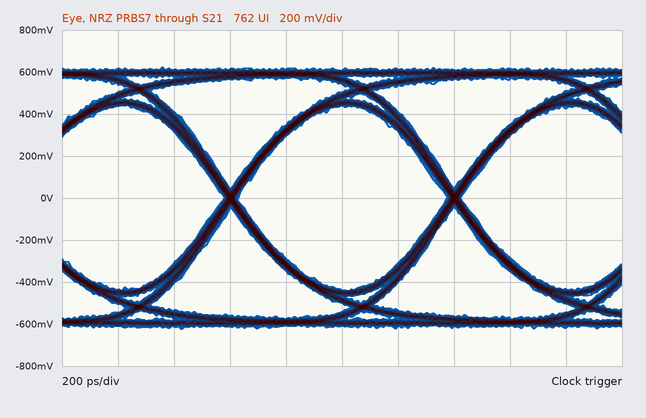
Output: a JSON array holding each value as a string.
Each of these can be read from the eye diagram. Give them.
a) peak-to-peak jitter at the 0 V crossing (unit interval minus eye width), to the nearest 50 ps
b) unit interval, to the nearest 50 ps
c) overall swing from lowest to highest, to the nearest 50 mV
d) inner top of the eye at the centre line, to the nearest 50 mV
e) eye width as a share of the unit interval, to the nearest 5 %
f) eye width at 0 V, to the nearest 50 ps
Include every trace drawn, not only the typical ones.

["50 ps", "800 ps", "1.25 V", "450 mV", "95 %", "750 ps"]
